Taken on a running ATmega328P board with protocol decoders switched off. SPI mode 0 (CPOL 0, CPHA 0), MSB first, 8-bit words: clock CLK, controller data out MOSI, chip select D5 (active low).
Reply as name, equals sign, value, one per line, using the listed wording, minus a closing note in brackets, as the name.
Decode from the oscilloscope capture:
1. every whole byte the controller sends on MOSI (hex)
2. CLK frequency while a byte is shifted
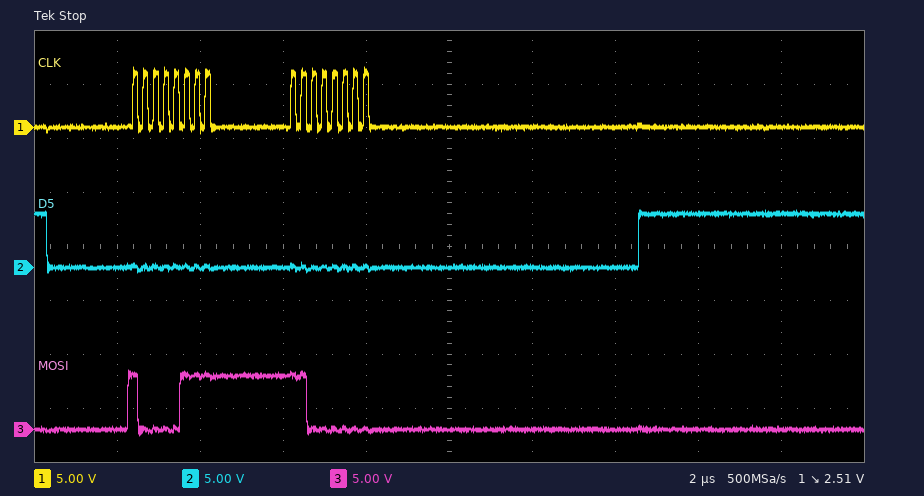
every whole byte the controller sends on MOSI = 0x87 0xC0
CLK frequency while a byte is shifted = 4 MHz
